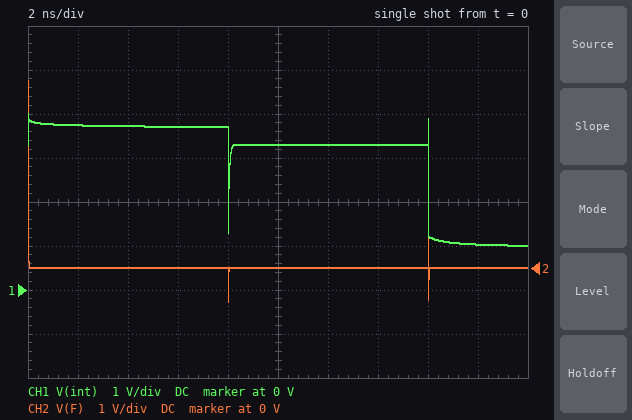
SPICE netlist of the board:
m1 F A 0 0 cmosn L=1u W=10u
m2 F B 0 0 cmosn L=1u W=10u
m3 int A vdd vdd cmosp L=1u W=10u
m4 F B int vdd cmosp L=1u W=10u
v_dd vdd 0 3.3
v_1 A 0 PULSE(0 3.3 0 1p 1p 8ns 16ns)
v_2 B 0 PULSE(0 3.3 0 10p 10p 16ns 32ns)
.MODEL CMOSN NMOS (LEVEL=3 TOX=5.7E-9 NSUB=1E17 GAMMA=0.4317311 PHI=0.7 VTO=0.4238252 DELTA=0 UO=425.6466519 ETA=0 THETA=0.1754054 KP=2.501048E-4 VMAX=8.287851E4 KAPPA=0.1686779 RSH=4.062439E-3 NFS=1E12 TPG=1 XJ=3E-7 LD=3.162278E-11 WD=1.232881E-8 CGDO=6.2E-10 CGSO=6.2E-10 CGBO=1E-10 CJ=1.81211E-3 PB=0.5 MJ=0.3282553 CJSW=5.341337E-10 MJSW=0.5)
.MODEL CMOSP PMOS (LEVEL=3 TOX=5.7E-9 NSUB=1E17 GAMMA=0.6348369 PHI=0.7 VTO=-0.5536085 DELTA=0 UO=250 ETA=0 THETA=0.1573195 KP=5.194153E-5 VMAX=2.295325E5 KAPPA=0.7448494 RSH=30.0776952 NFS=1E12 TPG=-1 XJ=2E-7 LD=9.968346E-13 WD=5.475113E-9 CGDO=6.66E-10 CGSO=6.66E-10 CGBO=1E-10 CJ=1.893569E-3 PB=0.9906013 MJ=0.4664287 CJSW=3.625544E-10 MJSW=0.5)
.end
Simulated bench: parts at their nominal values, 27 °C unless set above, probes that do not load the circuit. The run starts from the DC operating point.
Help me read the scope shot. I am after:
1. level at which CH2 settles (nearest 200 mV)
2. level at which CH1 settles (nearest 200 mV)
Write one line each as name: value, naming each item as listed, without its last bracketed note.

level at which CH2 settles: 0 V
level at which CH1 settles: 1.0 V
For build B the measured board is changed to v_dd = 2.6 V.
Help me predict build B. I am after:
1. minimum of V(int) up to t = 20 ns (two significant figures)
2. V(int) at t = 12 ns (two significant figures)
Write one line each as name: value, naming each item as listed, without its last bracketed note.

minimum of V(int) up to t = 20 ns: 810 mV
V(int) at t = 12 ns: 2.6 V
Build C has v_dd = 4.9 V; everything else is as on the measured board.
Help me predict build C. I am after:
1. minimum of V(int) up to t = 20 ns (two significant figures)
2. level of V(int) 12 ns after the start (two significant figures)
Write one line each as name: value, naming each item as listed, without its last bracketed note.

minimum of V(int) up to t = 20 ns: 2.1 V
level of V(int) 12 ns after the start: 4.8 V
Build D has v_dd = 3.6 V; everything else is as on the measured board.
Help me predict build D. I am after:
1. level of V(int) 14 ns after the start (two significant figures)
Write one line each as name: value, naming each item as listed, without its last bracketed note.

level of V(int) 14 ns after the start: 3.6 V
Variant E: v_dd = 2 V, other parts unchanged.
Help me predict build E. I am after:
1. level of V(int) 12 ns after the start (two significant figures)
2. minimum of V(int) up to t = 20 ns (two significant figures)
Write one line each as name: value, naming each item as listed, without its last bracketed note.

level of V(int) 12 ns after the start: 2.0 V
minimum of V(int) up to t = 20 ns: 670 mV
